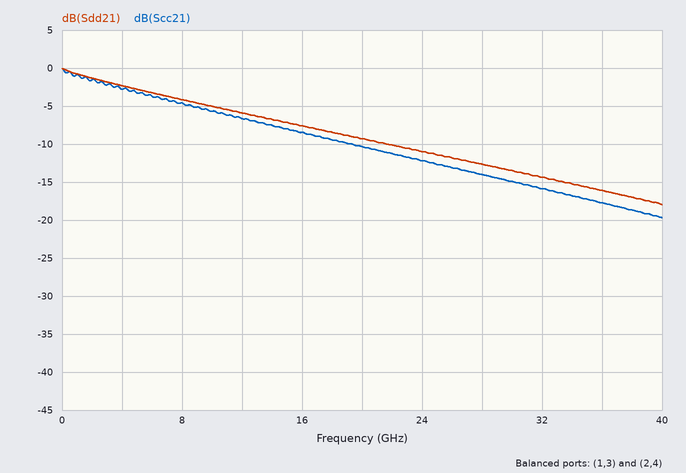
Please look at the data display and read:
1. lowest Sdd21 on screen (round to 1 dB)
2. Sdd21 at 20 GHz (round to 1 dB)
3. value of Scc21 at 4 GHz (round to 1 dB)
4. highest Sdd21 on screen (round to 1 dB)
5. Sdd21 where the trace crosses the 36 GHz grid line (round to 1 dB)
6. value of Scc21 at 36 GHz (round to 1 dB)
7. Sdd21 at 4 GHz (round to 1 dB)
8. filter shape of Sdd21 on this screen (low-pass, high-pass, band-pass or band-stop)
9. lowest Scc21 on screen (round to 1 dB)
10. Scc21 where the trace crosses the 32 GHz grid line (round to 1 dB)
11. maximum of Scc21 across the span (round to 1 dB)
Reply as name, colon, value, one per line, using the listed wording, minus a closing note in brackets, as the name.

lowest Sdd21 on screen: -18 dB
Sdd21 at 20 GHz: -9 dB
value of Scc21 at 4 GHz: -3 dB
highest Sdd21 on screen: 0 dB
Sdd21 where the trace crosses the 36 GHz grid line: -16 dB
value of Scc21 at 36 GHz: -18 dB
Sdd21 at 4 GHz: -2 dB
filter shape of Sdd21 on this screen: low-pass
lowest Scc21 on screen: -20 dB
Scc21 where the trace crosses the 32 GHz grid line: -16 dB
maximum of Scc21 across the span: 0 dB
